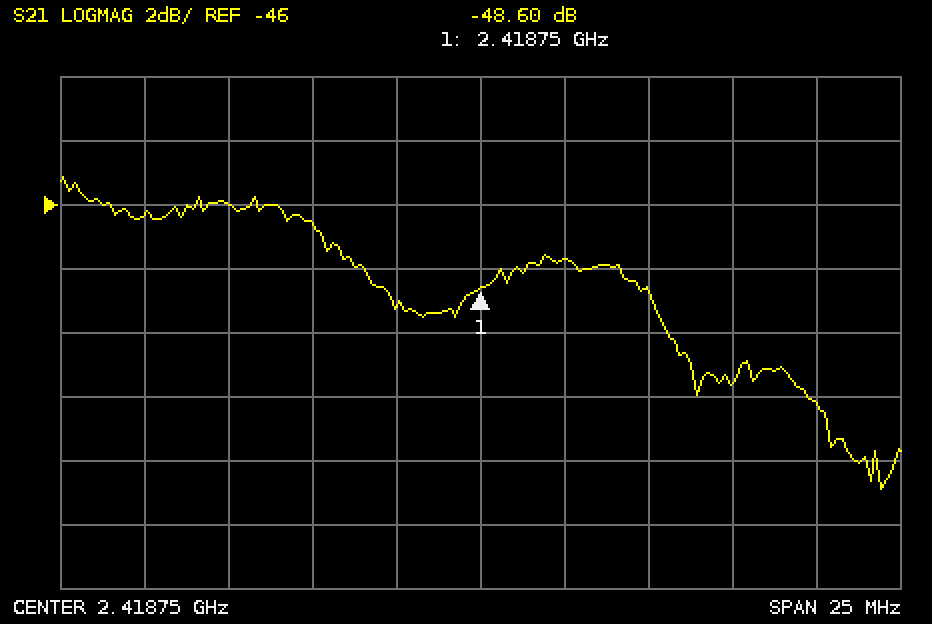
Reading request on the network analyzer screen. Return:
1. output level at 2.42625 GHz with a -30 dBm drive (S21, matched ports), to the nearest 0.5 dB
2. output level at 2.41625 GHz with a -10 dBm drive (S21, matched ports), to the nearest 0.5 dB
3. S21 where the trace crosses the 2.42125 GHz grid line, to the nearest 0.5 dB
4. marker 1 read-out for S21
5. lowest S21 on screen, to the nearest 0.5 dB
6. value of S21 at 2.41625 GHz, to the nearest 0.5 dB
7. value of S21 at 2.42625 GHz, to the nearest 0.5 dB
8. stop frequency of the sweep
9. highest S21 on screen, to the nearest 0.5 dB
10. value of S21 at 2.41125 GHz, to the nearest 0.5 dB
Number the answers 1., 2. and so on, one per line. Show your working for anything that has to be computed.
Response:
1. -30 dBm + (-51.5 dB) = -81.5 dBm
2. -10 dBm + (-49.0 dB) = -59.0 dBm
3. -47.5 dB
4. -48.60 dB
5. -55.0 dB
6. -49.0 dB
7. -51.5 dB
8. 2.43125 GHz
9. -45.0 dB
10. -46.0 dB
